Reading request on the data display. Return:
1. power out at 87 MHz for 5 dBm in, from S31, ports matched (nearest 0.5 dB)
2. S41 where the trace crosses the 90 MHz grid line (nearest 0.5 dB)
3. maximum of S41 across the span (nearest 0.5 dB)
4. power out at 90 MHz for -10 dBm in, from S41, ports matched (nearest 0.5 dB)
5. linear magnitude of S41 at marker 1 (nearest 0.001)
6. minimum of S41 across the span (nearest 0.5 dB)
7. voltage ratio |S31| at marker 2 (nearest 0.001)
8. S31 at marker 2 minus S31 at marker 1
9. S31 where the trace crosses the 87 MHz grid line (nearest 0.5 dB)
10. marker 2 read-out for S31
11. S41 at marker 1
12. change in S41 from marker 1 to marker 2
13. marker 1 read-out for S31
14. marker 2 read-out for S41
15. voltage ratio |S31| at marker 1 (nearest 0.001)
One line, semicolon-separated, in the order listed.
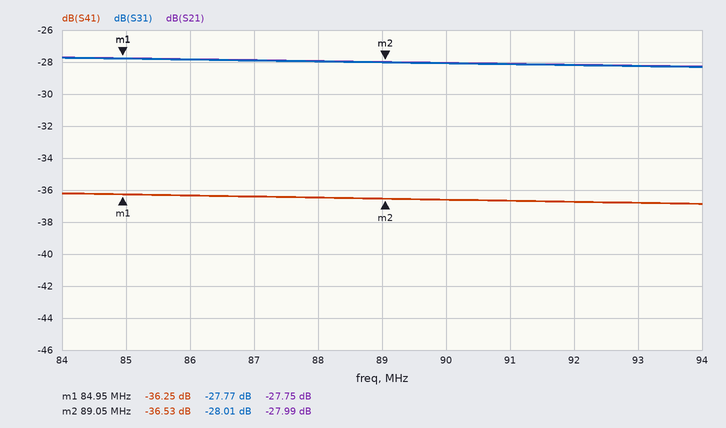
-23.0 dBm; -36.5 dB; -36.0 dB; -46.5 dBm; 0.015; -37.0 dB; 0.040; -0.24 dB; -28.0 dB; -28.01 dB; -36.25 dB; -0.28 dB; -27.77 dB; -36.53 dB; 0.041
